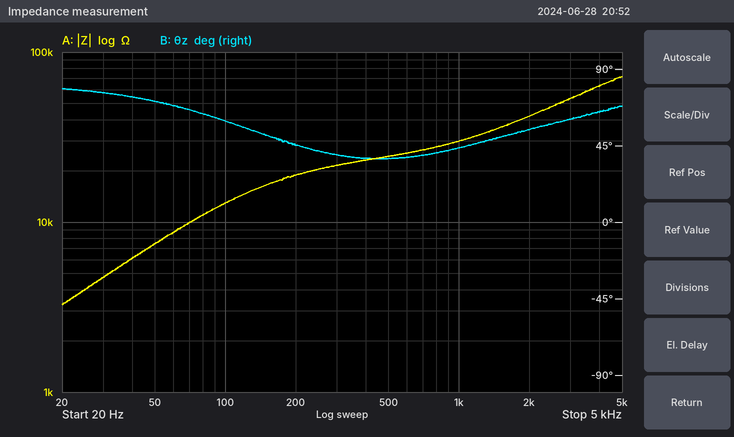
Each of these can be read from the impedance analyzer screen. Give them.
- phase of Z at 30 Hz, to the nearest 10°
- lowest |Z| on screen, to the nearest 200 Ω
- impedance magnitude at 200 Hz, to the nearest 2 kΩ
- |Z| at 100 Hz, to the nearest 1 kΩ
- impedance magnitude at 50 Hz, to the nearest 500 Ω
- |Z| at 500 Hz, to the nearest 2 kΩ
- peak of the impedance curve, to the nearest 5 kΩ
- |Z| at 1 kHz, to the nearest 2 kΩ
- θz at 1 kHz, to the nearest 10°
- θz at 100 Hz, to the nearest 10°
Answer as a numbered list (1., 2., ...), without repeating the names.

1. 80°
2. 3.2 kΩ
3. 18 kΩ
4. 13 kΩ
5. 7.5 kΩ
6. 24 kΩ
7. 70 kΩ
8. 30 kΩ
9. 40°
10. 60°
